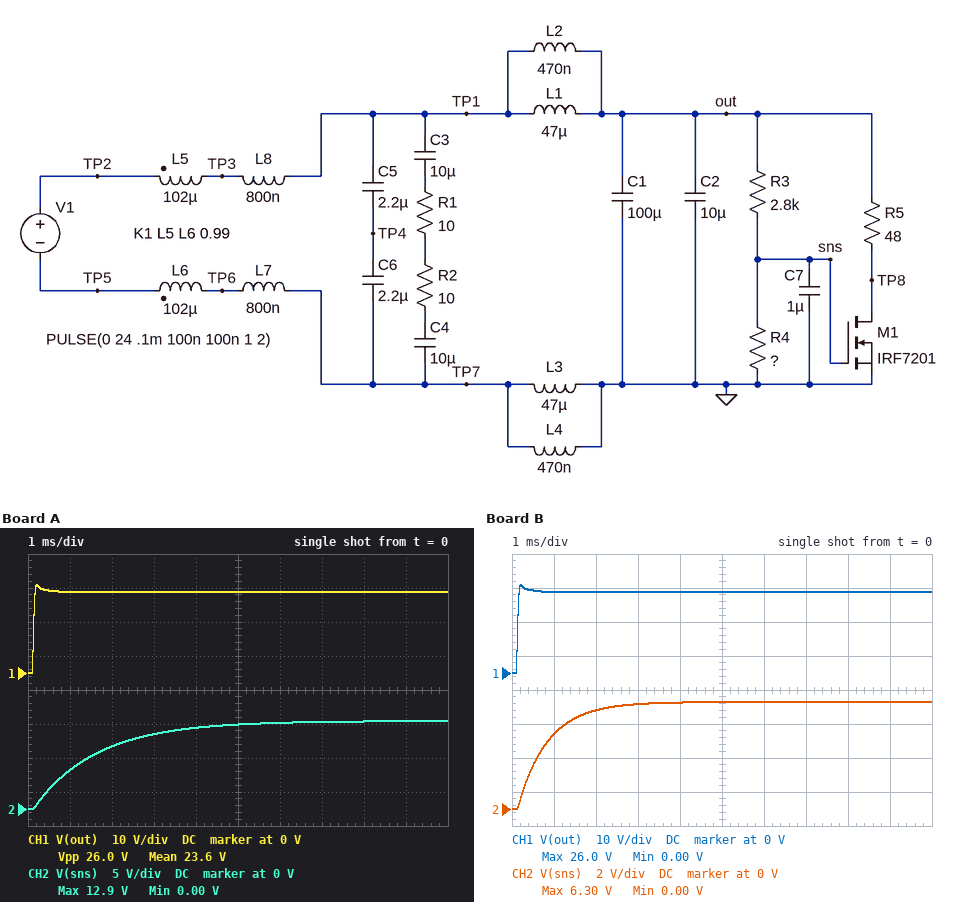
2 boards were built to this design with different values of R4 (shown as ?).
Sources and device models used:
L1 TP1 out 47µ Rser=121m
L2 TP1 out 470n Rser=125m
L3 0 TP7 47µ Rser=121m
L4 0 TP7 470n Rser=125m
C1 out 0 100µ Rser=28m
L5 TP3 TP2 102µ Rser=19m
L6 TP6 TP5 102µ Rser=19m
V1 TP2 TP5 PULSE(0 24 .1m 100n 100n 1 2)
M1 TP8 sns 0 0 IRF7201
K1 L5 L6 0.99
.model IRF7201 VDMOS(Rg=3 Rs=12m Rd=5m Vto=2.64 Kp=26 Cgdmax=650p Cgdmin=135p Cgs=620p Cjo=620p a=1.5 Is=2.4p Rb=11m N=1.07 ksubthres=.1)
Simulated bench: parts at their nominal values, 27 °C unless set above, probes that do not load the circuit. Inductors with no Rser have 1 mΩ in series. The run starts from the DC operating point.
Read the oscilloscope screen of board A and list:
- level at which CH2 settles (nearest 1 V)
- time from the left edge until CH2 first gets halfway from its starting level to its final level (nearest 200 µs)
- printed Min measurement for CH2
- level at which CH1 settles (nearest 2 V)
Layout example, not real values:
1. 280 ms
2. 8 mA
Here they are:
1. 13 V
2. 1.2 ms
3. 0.00 V
4. 24 V
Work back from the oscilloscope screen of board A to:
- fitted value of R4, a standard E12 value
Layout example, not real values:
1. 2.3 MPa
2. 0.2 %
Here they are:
1. 3.3 kΩ
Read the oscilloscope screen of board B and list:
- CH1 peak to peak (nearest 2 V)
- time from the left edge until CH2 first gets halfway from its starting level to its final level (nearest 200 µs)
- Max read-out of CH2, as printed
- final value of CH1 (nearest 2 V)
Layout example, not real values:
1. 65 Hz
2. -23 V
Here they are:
1. 26 V
2. 600 µs
3. 6.30 V
4. 24 V
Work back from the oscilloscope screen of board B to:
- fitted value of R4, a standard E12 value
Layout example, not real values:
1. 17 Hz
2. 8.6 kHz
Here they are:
1. 1 kΩ
